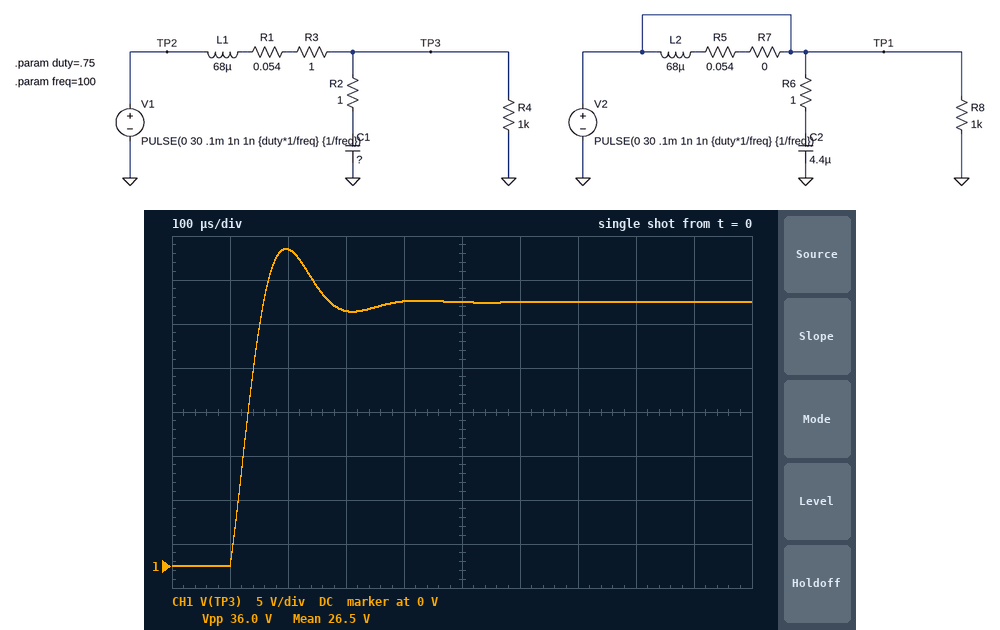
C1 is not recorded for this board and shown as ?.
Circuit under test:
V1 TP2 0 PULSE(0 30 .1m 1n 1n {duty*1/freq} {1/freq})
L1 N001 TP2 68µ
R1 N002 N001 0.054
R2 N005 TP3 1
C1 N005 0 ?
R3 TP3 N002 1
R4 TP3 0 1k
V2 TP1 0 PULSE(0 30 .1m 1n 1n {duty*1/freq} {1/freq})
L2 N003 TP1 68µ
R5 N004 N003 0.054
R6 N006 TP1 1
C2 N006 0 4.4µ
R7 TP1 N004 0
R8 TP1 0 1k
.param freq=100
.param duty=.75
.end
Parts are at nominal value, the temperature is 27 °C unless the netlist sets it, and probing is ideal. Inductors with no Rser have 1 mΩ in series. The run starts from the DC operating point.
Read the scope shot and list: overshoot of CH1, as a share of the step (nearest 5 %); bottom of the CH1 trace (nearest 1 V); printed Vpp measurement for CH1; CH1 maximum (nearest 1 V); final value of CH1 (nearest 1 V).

20 %
0 V
36.0 V
36 V
30 V
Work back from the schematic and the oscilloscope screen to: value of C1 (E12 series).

15 µF
